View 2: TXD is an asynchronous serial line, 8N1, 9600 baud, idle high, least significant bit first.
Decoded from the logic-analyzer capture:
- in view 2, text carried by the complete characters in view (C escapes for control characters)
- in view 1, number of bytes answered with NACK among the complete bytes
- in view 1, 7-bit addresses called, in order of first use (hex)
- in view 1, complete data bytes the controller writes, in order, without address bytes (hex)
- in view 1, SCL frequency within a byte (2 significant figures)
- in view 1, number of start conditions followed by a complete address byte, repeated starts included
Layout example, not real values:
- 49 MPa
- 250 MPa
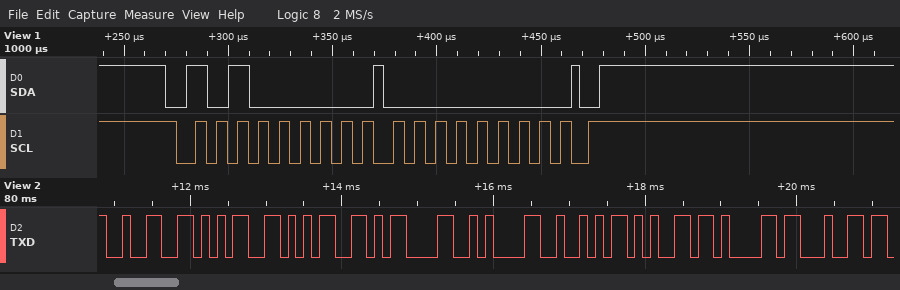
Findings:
- "255\r\nRead"
- 0
- 0x50
- 00
- 100 kHz
- 1
